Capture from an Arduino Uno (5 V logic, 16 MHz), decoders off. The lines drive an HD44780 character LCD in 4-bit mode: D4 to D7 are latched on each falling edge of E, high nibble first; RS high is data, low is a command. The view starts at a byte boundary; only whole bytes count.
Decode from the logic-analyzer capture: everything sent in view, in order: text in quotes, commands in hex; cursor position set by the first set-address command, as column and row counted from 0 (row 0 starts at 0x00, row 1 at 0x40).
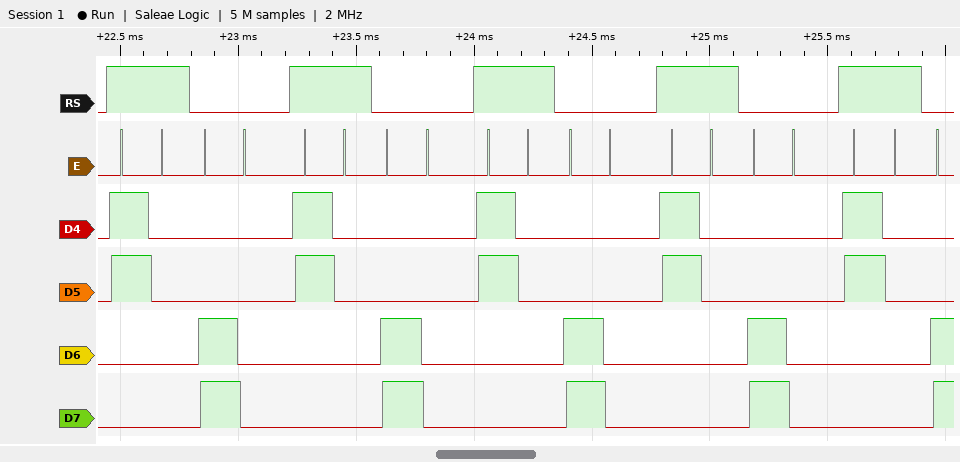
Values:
"0" 0xC0 "0" 0xC0 "0" 0xC0 "0" 0xC0 "0"
column 0, row 1
